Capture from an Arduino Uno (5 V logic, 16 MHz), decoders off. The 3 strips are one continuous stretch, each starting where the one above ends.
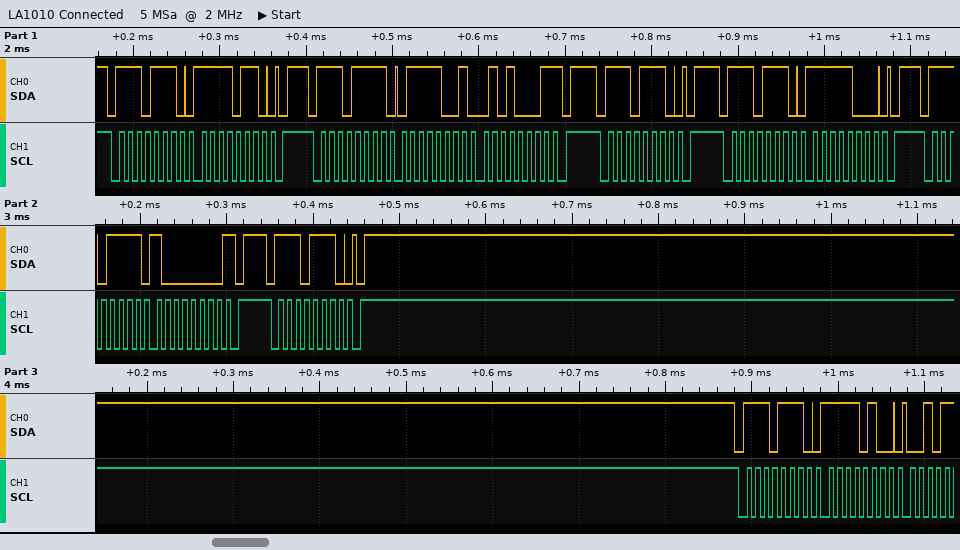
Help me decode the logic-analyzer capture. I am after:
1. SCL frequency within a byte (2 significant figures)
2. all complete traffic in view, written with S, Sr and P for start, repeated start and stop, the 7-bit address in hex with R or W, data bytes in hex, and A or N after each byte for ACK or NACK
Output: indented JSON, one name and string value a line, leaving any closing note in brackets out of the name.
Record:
{
  "SCL frequency within a byte": "100 kHz",
  "all complete traffic in view, written with S, Sr and P for start, repeated start and stop, the 7-bit address in hex with R or W, data bytes in hex, and A or N after each byte for ACK or NACK": "S 77W A F6 A P S 77R A 79 A 51 N P S 77W A P S 77W A F8 A P S 77R A 80 N P S 77W A P S 77W A F4 A"
}
